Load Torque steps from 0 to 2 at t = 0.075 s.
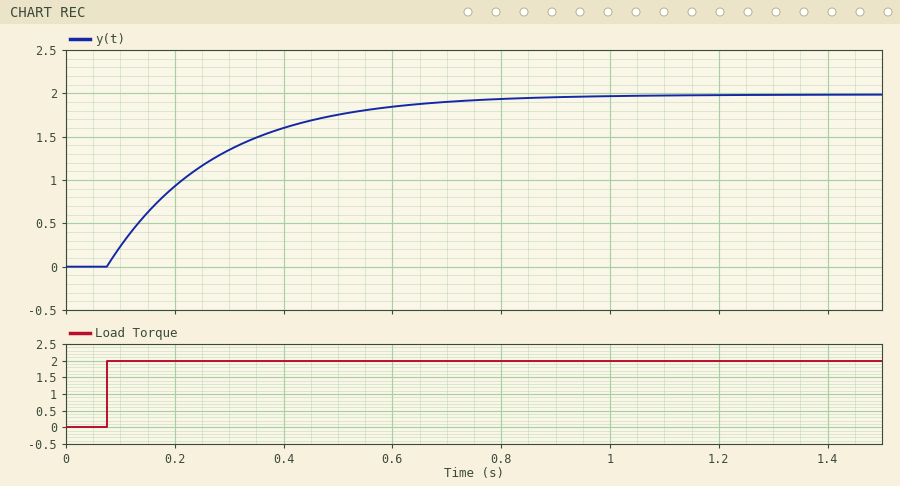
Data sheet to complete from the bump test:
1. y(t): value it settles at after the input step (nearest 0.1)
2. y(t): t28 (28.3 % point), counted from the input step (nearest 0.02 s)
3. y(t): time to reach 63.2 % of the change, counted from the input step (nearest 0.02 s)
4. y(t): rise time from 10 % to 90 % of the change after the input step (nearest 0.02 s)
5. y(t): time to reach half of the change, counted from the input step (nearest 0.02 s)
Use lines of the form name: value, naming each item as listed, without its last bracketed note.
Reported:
y(t): value it settles at after the input step: 2.0
y(t): t28 (28.3 % point), counted from the input step: 0.06 s
y(t): time to reach 63.2 % of the change, counted from the input step: 0.20 s
y(t): rise time from 10 % to 90 % of the change after the input step: 0.44 s
y(t): time to reach half of the change, counted from the input step: 0.14 s
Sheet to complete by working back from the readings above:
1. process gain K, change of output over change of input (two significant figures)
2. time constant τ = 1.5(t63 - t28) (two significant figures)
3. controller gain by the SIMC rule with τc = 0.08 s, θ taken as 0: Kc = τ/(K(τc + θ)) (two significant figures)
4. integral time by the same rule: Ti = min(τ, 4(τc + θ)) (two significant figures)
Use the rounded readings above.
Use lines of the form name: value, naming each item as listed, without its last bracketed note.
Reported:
process gain K, change of output over change of input: 1.0
time constant τ = 1.5(t63 - t28): 0.21 s
controller gain by the SIMC rule with τc = 0.08 s, θ taken as 0: Kc = τ/(K(τc + θ)): 2.6
integral time by the same rule: Ti = min(τ, 4(τc + θ)): 0.21 s
